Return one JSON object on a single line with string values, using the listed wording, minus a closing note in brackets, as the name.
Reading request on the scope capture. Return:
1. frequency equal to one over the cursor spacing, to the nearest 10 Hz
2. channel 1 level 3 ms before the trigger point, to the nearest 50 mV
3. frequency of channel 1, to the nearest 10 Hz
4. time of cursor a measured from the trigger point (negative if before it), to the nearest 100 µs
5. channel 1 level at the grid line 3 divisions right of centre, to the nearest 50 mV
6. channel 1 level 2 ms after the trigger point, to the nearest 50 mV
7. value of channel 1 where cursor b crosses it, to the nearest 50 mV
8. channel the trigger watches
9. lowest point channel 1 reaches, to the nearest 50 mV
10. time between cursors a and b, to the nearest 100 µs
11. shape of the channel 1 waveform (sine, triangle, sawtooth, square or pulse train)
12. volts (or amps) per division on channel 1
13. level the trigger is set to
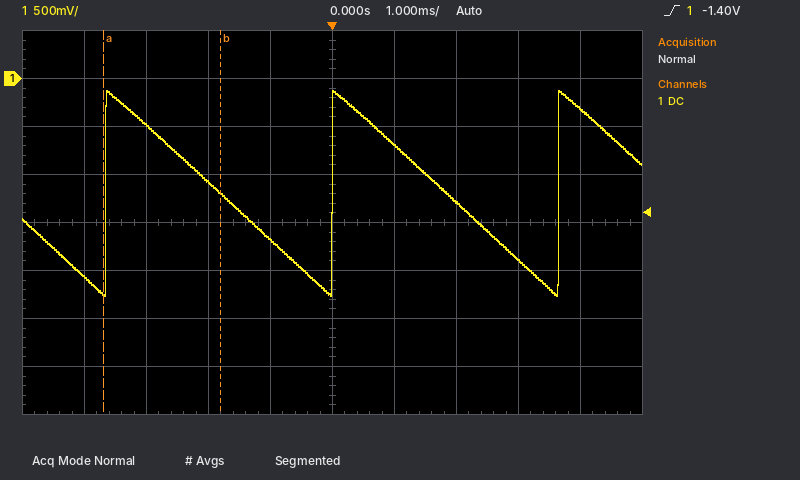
{"frequency equal to one over the cursor spacing, to the nearest 10 Hz": "530 Hz", "channel 1 level 3 ms before the trigger point, to the nearest 50 mV": "-500 mV", "frequency of channel 1, to the nearest 10 Hz": "270 Hz", "time of cursor a measured from the trigger point (negative if before it), to the nearest 100 µs": "-3.7 ms", "channel 1 level at the grid line 3 divisions right of centre, to the nearest 50 mV": "-1.90 V", "channel 1 level 2 ms after the trigger point, to the nearest 50 mV": "-1.30 V", "value of channel 1 where cursor b crosses it, to the nearest 50 mV": "-1.20 V", "channel the trigger watches": "channel 1", "lowest point channel 1 reaches, to the nearest 50 mV": "-2.25 V", "time between cursors a and b, to the nearest 100 µs": "1.9 ms", "shape of the channel 1 waveform": "sawtooth", "volts (or amps) per division on channel 1": "500 mV", "level the trigger is set to": "-1.40 V"}
